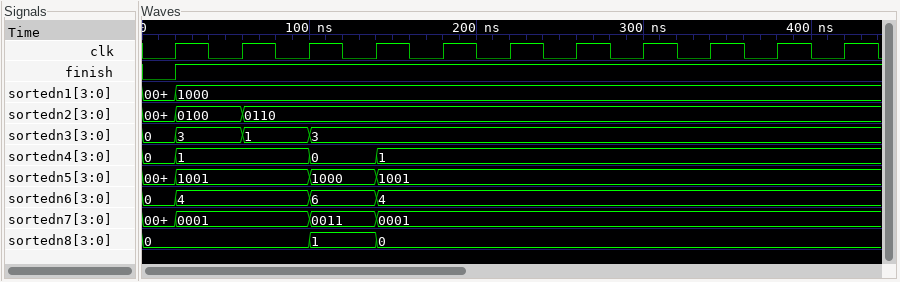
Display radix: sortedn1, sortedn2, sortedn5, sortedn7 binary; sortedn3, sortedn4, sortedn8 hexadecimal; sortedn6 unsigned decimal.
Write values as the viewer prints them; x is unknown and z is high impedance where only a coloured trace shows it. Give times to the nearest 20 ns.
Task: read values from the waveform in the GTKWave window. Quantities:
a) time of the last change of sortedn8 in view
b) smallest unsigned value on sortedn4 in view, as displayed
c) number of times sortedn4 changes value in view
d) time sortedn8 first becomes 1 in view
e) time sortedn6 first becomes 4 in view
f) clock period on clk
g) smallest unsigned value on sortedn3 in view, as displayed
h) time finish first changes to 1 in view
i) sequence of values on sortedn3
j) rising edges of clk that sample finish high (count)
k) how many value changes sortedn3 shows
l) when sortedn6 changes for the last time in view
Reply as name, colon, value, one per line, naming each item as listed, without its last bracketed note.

time of the last change of sortedn8 in view: 140 ns
smallest unsigned value on sortedn4 in view, as displayed: 0
number of times sortedn4 changes value in view: 3
time sortedn8 first becomes 1 in view: 100 ns
time sortedn6 first becomes 4 in view: 20 ns
clock period on clk: 40 ns
smallest unsigned value on sortedn3 in view, as displayed: 0
time finish first changes to 1 in view: 20 ns
sequence of values on sortedn3: 0, 3, 1, 3
rising edges of clk that sample finish high: 10
how many value changes sortedn3 shows: 3
when sortedn6 changes for the last time in view: 140 ns
